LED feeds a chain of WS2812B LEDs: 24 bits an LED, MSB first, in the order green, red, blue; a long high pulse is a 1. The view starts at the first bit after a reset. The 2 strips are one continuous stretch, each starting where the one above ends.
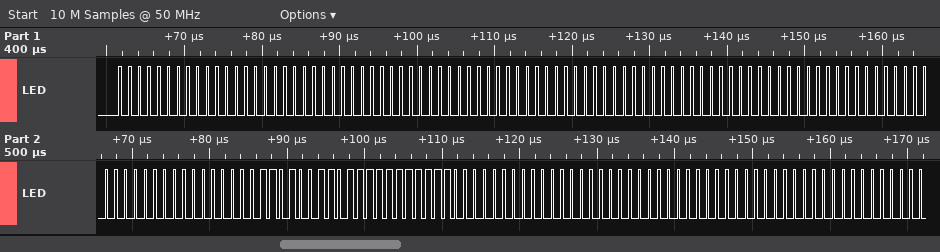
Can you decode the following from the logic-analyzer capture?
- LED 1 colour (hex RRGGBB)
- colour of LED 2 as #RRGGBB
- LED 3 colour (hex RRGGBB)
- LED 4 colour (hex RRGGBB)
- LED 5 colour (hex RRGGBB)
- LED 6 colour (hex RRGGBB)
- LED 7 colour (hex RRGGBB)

#000000
#000000
#000000
#000000
#370DFF
#000000
#000000
